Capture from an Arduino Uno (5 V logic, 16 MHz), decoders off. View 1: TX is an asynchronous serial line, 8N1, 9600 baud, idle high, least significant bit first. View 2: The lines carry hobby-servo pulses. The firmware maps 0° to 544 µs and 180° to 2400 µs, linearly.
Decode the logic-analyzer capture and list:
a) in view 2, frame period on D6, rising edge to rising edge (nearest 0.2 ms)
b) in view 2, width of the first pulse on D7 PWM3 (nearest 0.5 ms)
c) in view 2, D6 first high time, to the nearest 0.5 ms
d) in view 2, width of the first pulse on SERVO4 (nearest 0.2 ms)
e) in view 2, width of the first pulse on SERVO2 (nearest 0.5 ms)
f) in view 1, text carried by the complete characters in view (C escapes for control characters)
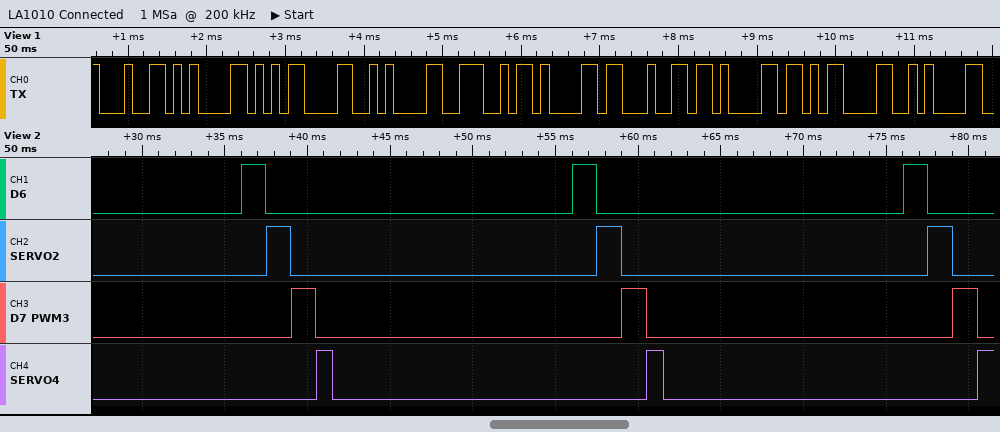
20.0 ms
1.5 ms
1.5 ms
1.0 ms
1.5 ms
"da\r\nNada\r\n"
